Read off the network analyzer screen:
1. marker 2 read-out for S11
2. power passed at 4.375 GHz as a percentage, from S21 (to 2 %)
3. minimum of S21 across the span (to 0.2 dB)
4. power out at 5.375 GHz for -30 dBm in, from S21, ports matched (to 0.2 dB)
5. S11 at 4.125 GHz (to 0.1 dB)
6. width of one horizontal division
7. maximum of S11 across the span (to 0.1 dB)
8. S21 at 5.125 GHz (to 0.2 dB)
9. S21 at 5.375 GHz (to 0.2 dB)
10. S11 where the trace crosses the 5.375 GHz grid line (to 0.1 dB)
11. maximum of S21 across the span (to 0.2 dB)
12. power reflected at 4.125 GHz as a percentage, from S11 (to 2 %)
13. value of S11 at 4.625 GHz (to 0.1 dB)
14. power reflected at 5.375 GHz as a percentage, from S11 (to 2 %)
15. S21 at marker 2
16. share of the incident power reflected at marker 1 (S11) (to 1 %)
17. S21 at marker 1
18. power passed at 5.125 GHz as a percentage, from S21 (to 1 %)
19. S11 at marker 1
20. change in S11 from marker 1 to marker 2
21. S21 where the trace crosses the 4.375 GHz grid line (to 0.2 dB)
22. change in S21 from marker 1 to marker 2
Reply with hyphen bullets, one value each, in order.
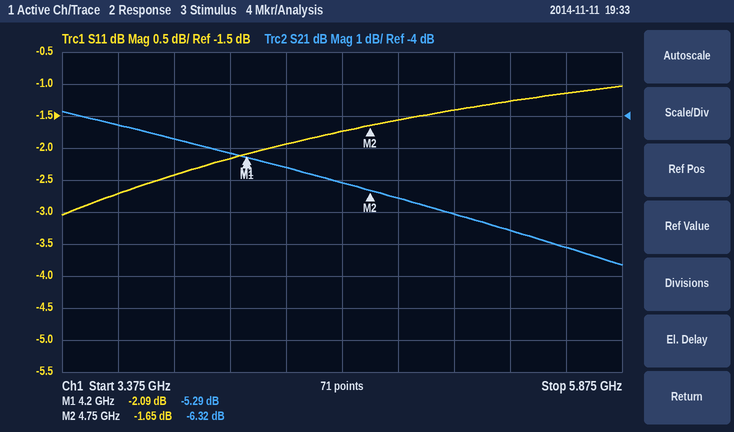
- -1.65 dB
- 28 %
- -8.6 dB
- -37.6 dBm
- -2.2 dB
- 250 MHz
- -1.0 dB
- -7.0 dB
- -7.6 dB
- -1.3 dB
- -3.8 dB
- 60 %
- -1.7 dB
- 74 %
- -6.32 dB
- 62 %
- -5.29 dB
- 20 %
- -2.09 dB
- 0.44 dB
- -5.6 dB
- -1.03 dB
